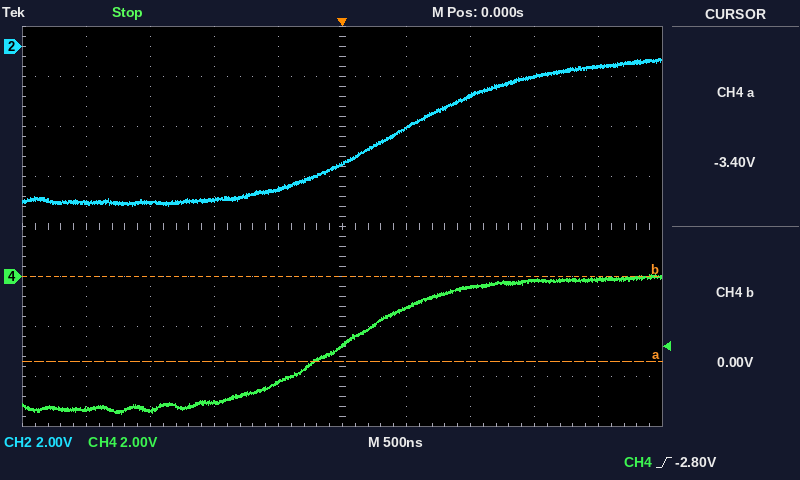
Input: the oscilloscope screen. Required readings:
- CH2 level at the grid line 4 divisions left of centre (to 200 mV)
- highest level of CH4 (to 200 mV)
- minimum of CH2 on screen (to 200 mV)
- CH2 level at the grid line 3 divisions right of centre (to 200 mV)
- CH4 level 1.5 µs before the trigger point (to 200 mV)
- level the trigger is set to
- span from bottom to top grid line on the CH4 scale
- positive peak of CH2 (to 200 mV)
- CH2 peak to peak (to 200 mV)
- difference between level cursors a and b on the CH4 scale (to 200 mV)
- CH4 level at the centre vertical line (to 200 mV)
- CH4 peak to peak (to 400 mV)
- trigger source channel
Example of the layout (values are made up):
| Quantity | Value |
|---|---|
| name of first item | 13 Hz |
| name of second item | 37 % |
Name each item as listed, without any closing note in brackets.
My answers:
| Quantity | Value |
|---|---|
| CH2 level at the grid line 4 divisions left of centre | -6.2 V |
| highest level of CH4 | 0.0 V |
| minimum of CH2 on screen | -6.4 V |
| CH2 level at the grid line 3 divisions right of centre | -1.2 V |
| CH4 level 1.5 µs before the trigger point | -5.4 V |
| level the trigger is set to | -2.80 V |
| span from bottom to top grid line on the CH4 scale | 16 V |
| positive peak of CH2 | -400 mV |
| CH2 peak to peak | 6.0 V |
| difference between level cursors a and b on the CH4 scale | 3.4 V |
| CH4 level at the centre vertical line | -2.8 V |
| CH4 peak to peak | 5.6 V |
| trigger source channel | CH4 |
